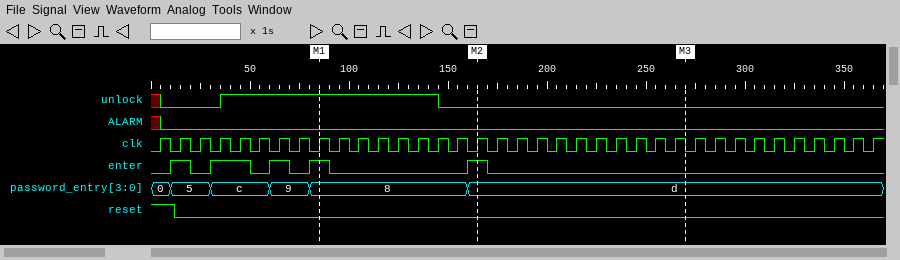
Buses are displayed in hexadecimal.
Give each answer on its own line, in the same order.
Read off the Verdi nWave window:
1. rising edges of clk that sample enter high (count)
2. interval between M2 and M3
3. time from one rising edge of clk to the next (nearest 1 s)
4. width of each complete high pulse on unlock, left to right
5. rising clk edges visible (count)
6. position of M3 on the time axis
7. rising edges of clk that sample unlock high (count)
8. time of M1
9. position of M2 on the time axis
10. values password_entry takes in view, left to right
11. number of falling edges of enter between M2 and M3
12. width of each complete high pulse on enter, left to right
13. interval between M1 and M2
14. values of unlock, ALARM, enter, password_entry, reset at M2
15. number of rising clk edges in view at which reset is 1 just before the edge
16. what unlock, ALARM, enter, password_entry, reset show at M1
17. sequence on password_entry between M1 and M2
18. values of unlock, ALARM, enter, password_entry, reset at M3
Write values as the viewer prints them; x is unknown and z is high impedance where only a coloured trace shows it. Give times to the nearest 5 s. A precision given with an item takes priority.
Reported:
6
105 s
10 s
110 s
37
270 s
11
85 s
165 s
0, 5, c, 9, 8, d
1
10 s, 20 s, 10 s, 10 s, 10 s
80 s
unlock=0, ALARM=0, enter=1, password_entry=d, reset=0
1
unlock=1, ALARM=0, enter=1, password_entry=8, reset=0
8, d
unlock=0, ALARM=0, enter=0, password_entry=d, reset=0
